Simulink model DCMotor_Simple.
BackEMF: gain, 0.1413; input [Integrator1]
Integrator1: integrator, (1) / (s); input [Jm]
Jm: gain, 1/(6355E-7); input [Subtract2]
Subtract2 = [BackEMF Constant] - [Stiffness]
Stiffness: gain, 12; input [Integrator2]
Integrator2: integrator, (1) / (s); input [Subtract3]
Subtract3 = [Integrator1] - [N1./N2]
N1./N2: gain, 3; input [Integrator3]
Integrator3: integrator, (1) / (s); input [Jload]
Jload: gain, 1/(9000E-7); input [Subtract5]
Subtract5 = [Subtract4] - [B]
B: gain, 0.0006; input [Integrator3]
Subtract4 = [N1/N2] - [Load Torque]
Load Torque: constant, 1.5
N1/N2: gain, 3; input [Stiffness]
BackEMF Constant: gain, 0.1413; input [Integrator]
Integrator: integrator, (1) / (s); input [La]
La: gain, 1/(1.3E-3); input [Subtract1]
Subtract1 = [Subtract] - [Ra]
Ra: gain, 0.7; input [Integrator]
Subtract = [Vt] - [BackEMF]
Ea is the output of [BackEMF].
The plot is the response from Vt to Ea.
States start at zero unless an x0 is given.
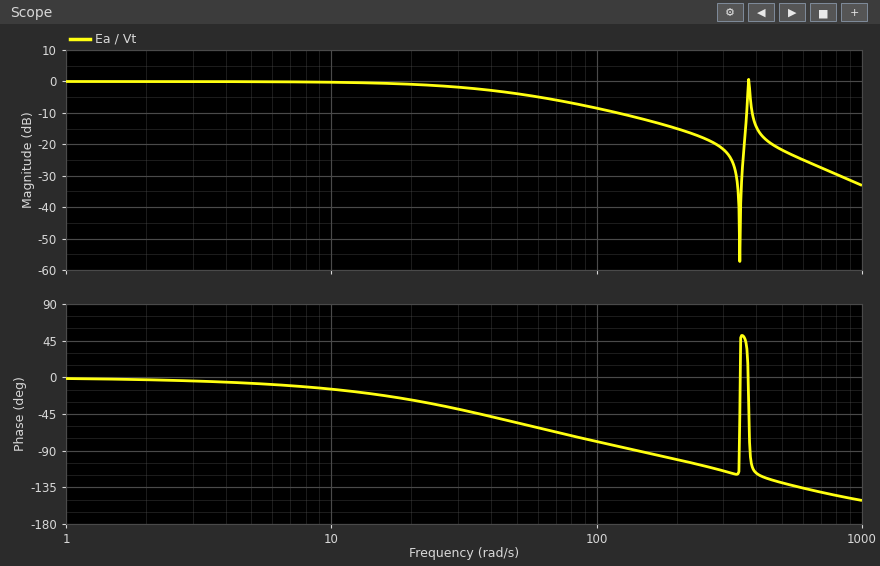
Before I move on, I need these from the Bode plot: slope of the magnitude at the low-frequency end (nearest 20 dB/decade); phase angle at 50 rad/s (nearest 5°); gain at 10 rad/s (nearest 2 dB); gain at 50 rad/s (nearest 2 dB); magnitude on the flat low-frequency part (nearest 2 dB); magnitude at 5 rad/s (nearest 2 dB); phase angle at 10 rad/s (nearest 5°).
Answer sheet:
0 dB/decade
-55°
0 dB
-4 dB
0 dB
0 dB
-15°
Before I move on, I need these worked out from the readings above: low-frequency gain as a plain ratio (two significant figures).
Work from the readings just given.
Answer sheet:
1.0
